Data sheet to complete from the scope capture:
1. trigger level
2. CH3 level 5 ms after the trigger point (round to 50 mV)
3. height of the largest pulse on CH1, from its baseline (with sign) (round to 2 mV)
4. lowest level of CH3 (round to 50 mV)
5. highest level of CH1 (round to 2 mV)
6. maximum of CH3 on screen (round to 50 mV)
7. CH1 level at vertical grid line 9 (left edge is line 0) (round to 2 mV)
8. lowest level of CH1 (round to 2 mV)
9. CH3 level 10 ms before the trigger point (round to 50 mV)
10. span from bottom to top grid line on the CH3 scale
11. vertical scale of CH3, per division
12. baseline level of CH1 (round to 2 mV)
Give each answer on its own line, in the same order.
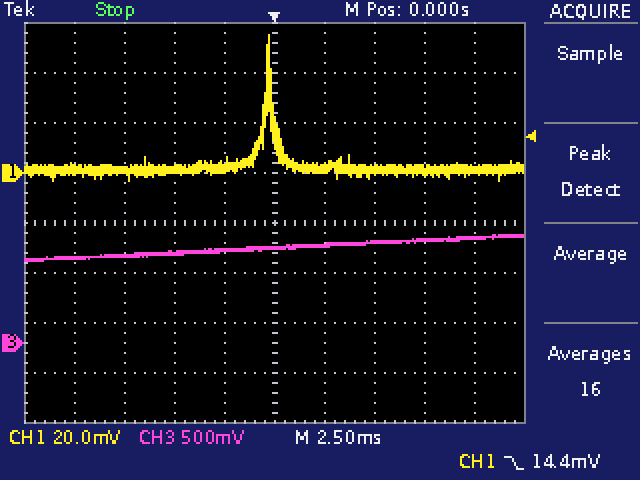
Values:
14.4 mV
1.00 V
+54 mV
800 mV
56 mV
1.10 V
2 mV
-4 mV
850 mV
4 V
500 mV
2 mV
